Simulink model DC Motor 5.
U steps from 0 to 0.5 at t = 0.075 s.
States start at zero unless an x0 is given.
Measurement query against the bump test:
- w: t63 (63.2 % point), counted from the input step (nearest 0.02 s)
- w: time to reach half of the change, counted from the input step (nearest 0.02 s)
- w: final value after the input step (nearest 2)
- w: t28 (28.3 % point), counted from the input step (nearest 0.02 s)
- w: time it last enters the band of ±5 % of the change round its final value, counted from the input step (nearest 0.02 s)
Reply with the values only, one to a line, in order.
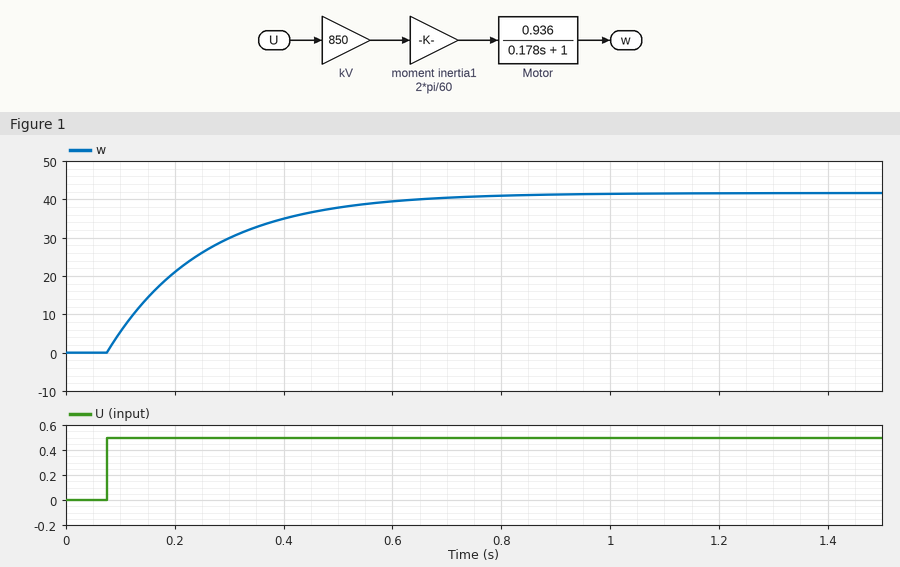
0.18 s
0.12 s
42
0.06 s
0.54 s
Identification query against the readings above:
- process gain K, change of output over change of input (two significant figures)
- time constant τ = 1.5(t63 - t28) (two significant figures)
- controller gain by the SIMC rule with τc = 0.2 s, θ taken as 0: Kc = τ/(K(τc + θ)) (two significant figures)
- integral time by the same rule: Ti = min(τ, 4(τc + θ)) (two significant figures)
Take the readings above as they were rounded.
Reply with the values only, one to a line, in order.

84
0.18 s
0.011
0.18 s
